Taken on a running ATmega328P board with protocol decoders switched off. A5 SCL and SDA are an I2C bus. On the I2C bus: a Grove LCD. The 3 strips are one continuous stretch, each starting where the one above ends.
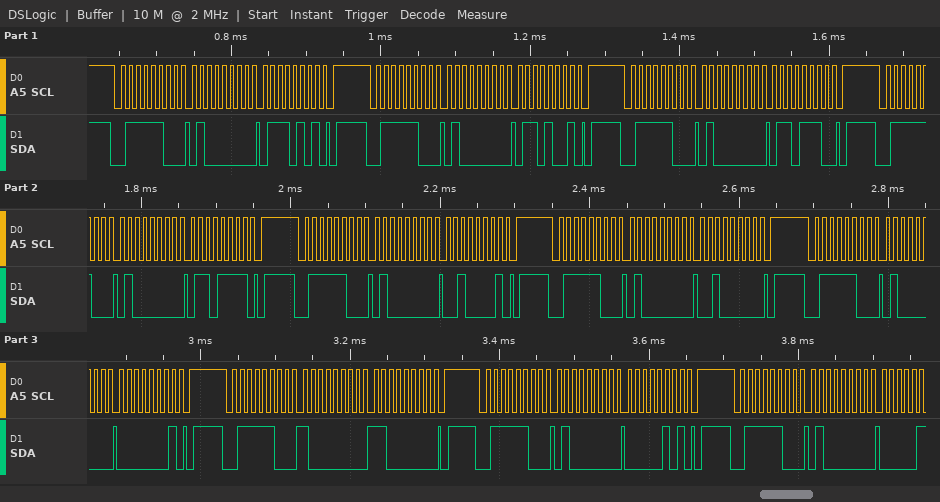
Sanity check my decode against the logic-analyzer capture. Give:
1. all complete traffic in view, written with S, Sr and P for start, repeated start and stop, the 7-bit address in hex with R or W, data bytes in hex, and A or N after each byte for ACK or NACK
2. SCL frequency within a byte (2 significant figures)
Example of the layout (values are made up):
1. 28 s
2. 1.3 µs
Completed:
1. S 3EW A 40 A 75 A P S 3EW A 40 A 69 A P S 3EW A 40 A 6E A P S 3EW A 40 A 6F A P S 3EW A 40 A 21 A P S 3EW A 40 A 20 A P S 3EW A 40 A 01 A P S 3EW A 80 A C0 A P S 3EW A 40 A 05 A P S 3EW A 40 A
2. 100 kHz
